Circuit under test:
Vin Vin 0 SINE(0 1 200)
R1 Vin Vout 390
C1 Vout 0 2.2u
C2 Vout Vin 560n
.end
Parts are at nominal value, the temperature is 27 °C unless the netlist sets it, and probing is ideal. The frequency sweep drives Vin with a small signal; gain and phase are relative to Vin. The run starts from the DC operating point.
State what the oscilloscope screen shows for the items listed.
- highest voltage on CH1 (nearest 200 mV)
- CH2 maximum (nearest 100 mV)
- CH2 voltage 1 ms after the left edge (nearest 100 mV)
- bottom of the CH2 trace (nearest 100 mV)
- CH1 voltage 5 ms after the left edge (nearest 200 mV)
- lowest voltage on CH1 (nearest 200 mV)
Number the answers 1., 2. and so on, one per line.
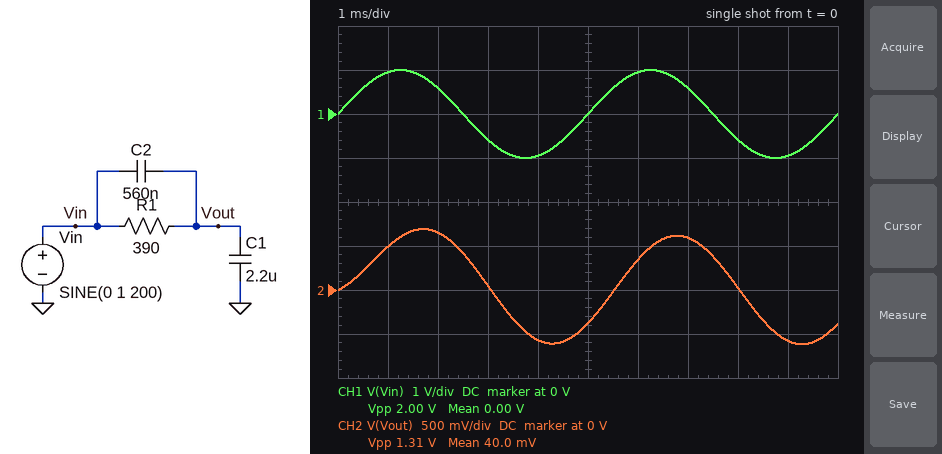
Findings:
1. 1.0 V
2. 700 mV
3. 500 mV
4. -600 mV
5. 0 V
6. -1.0 V
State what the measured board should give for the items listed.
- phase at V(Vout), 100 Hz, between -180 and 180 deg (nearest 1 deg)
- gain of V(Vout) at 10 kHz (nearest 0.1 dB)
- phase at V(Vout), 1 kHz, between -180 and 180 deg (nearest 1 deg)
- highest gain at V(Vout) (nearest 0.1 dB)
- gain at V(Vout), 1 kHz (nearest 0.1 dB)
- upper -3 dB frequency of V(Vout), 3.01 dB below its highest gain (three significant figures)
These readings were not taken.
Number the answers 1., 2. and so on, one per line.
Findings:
1. -26 deg
2. -13.8 dB
3. -28 deg
4. 0 dB
5. -12.1 dB
6. 154 Hz
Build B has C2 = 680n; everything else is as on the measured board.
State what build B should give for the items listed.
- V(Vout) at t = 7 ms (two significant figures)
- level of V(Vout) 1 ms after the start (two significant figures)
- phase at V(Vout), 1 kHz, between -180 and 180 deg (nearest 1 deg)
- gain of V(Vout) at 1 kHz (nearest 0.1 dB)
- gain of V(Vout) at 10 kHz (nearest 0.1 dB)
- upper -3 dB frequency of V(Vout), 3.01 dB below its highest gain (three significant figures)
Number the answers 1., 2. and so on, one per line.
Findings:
1. 580 mV
2. 500 mV
3. -23 deg
4. -11.3 dB
5. -12.5 dB
6. 150 Hz
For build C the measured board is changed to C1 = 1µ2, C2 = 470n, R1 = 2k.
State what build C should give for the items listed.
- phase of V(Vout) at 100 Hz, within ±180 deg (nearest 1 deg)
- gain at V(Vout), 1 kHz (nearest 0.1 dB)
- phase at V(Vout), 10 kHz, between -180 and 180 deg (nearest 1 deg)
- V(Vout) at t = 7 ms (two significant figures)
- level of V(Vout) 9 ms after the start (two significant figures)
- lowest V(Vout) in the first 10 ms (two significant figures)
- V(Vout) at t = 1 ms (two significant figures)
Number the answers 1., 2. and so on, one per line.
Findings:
1. -34 deg
2. -10.9 dB
3. -1 deg
4. 340 mV
5. -340 mV
6. -350 mV
7. 370 mV
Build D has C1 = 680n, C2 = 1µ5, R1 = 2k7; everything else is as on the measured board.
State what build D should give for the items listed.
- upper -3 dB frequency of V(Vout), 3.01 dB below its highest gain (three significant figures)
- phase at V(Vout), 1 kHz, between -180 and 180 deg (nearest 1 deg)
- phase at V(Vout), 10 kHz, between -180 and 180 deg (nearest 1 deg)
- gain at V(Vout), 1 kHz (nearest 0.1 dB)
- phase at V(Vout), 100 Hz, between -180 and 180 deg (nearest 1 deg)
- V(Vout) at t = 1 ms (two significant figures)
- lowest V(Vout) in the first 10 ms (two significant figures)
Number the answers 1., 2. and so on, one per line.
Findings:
1. 117 Hz
2. -1 deg
3. 0 deg
4. -3.2 dB
5. -6 deg
6. 680 mV
7. -690 mV
